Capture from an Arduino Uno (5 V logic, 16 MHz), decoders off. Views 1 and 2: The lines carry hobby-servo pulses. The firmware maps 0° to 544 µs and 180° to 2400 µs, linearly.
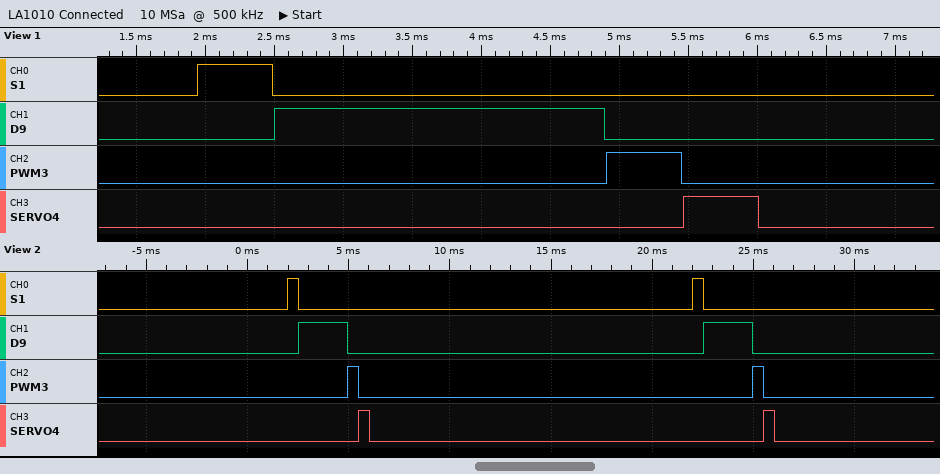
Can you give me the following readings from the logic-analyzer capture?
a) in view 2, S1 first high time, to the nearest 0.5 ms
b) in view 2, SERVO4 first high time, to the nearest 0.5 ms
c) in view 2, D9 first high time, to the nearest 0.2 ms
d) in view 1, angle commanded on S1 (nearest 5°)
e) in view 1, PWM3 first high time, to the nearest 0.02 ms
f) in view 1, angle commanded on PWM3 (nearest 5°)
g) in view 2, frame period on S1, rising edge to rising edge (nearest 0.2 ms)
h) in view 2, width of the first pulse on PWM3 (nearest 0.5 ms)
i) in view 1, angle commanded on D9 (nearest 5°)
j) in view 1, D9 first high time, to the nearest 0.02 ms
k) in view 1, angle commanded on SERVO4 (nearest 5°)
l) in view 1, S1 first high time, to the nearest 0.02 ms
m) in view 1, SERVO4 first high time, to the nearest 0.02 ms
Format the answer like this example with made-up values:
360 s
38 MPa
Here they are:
0.5 ms
0.5 ms
2.4 ms
0°
0.54 ms
0°
20.0 ms
0.5 ms
180°
2.40 ms
0°
0.54 ms
0.54 ms
